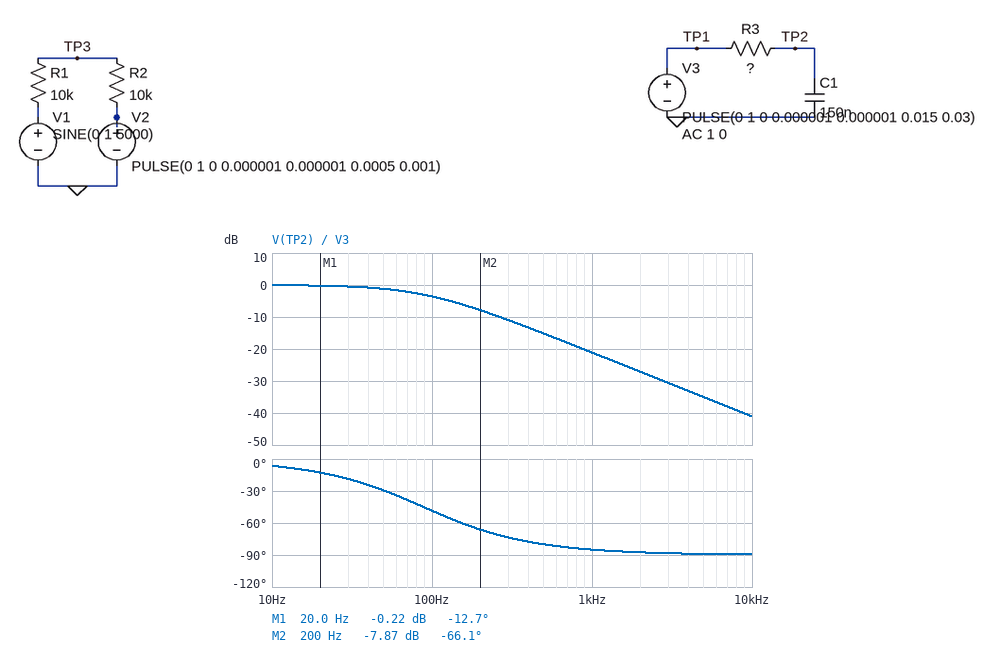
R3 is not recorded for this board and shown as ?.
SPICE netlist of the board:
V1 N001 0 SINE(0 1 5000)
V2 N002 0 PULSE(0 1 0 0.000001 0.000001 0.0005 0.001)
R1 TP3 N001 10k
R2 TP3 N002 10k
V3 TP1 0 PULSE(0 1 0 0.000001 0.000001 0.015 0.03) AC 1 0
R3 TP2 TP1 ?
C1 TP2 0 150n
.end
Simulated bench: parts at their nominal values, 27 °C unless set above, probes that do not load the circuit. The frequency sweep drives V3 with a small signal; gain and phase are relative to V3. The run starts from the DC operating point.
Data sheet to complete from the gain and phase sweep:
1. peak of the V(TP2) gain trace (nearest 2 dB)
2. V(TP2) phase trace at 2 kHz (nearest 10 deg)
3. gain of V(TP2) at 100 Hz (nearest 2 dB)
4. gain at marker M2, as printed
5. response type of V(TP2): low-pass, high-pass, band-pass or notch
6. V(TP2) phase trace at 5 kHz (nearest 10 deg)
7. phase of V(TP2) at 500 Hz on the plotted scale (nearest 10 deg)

0 dB
-90 deg
-4 dB
-7.87 dB
low-pass
-90 deg
-80 deg
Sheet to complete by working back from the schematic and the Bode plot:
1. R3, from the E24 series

12 kΩ
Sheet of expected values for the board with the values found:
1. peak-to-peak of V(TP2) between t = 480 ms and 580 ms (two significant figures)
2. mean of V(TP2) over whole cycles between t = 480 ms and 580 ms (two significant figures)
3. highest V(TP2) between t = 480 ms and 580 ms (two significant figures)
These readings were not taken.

1.0 V
500 mV
1.0 V
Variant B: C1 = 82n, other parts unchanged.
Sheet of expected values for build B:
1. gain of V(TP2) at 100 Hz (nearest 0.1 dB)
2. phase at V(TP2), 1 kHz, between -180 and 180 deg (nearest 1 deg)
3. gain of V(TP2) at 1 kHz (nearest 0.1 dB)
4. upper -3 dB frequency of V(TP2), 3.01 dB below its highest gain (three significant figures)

-1.4 dB
-81 deg
-15.9 dB
162 Hz
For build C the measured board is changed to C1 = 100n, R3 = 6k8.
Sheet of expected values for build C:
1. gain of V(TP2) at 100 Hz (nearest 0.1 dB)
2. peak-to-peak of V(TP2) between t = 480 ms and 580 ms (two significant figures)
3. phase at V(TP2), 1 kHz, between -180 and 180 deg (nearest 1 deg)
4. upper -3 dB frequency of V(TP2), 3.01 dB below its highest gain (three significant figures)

-0.7 dB
1.0 V
-77 deg
234 Hz
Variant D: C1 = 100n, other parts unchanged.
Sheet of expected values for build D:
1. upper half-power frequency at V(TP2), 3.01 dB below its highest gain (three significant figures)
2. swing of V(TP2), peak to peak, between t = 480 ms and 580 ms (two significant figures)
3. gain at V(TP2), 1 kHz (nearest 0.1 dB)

133 Hz
1.0 V
-17.6 dB
